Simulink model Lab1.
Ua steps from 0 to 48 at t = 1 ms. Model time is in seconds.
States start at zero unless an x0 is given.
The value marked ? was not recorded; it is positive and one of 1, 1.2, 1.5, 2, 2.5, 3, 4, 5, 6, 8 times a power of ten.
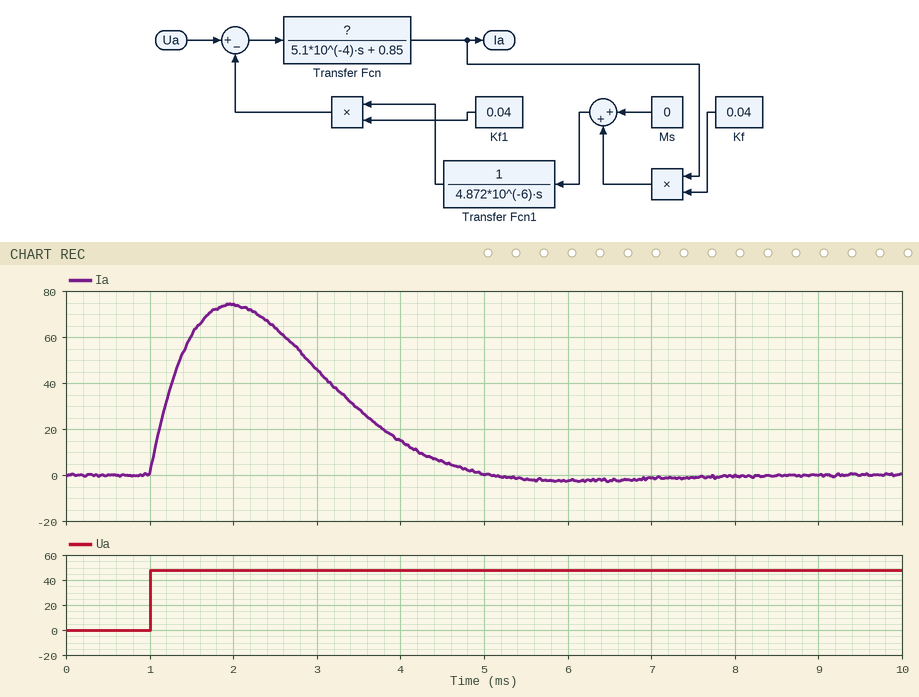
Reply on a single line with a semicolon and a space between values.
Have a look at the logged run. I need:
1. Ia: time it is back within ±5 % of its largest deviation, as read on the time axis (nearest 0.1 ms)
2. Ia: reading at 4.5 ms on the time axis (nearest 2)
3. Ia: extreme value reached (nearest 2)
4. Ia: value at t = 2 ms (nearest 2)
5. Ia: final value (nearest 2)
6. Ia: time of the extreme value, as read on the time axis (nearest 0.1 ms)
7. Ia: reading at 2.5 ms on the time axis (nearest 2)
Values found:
4.7 ms; 6; 74; 74; 0; 2.0 ms; 64
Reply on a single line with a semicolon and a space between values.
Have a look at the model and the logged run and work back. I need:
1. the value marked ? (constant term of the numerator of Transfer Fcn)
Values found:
2
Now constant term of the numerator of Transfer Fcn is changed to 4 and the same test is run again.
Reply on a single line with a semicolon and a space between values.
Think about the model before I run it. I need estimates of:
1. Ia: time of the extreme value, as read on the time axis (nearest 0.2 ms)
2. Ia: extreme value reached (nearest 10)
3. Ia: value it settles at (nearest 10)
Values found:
1.8 ms; 130; 0
